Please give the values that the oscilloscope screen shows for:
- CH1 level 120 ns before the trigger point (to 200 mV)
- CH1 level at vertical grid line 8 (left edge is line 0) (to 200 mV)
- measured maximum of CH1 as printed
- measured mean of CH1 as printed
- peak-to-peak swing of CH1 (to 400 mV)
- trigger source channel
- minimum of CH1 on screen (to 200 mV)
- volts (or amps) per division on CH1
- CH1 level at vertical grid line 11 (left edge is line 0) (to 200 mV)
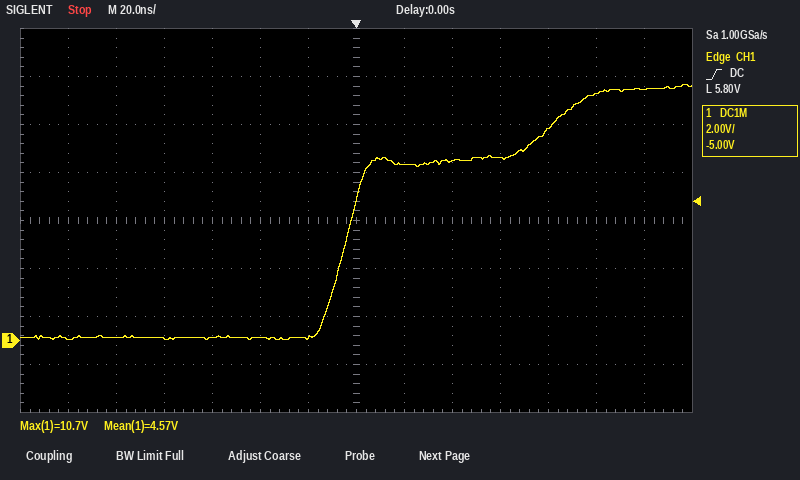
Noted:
0.0 V
7.4 V
10.7 V
4.57 V
10.8 V
CH1
0.0 V
2 V
8.8 V
